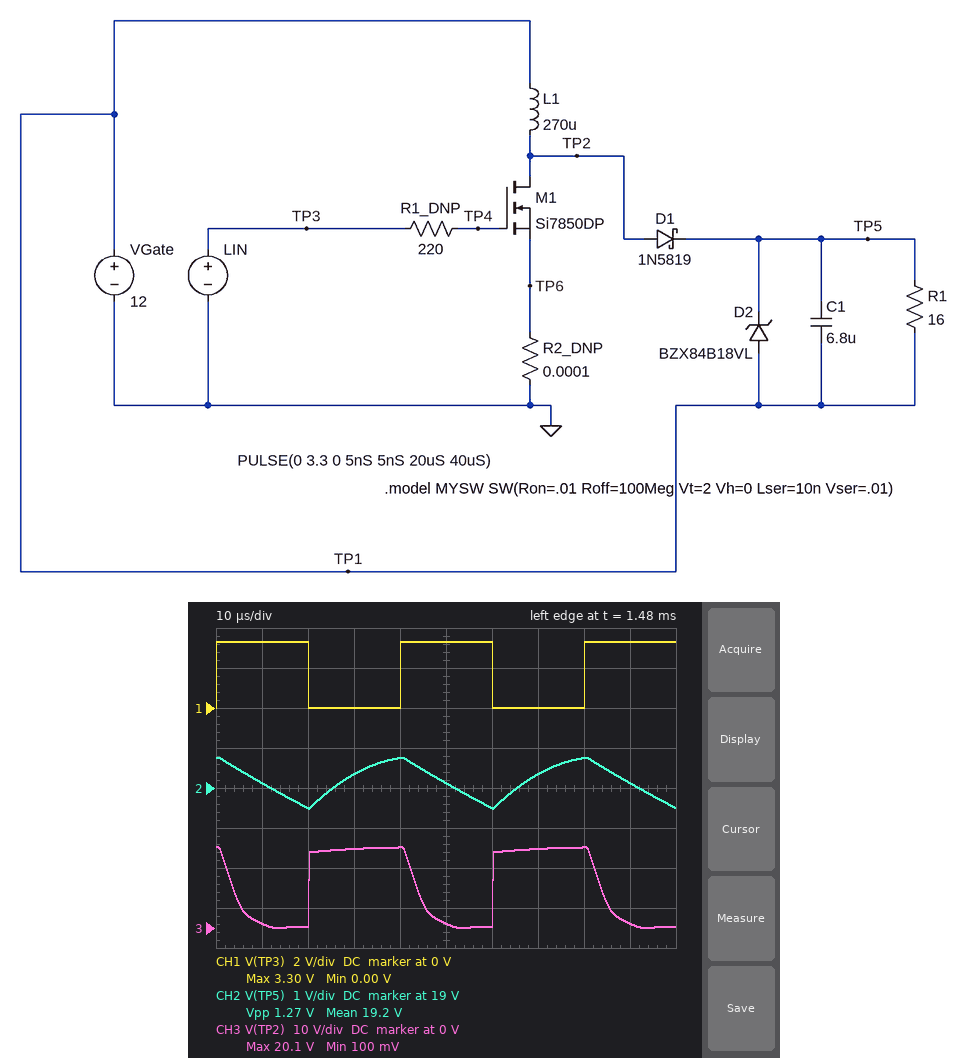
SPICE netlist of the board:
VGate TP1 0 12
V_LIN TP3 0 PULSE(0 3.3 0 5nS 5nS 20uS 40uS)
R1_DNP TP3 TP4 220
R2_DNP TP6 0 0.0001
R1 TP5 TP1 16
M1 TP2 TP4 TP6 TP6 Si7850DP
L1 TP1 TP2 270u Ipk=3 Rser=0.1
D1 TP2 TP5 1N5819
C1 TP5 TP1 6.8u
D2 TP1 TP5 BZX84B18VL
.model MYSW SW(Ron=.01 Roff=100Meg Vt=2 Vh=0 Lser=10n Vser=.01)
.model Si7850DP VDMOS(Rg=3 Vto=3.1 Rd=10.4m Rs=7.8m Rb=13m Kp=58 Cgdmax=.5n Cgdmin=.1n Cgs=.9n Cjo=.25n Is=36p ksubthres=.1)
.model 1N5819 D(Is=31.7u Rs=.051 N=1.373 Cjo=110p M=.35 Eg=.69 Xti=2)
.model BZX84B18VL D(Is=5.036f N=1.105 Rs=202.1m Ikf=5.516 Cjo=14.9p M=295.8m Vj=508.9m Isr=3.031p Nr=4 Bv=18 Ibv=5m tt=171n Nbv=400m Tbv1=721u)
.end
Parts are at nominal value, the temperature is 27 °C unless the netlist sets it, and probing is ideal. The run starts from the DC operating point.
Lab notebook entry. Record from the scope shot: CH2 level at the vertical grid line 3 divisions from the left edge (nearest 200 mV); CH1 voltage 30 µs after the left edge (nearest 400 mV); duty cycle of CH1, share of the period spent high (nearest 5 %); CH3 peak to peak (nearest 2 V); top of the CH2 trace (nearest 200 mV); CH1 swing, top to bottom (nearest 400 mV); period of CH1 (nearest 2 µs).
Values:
19.4 V
0 V
50 %
20 V
19.8 V
3.2 V
40 µs
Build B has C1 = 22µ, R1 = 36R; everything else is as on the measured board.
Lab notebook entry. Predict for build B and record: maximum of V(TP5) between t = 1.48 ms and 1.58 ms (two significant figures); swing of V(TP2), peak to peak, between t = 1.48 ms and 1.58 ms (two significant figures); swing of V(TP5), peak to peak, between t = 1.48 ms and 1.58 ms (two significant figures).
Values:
21 V
22 V
240 mV
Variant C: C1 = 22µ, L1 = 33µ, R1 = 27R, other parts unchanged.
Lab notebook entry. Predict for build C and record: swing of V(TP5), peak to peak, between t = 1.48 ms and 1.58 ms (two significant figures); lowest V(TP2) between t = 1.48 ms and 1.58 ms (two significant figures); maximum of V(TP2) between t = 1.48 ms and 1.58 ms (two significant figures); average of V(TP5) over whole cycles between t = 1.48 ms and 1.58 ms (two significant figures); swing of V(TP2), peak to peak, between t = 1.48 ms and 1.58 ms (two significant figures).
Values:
240 mV
1.5 V
18 V
17 V
16 V
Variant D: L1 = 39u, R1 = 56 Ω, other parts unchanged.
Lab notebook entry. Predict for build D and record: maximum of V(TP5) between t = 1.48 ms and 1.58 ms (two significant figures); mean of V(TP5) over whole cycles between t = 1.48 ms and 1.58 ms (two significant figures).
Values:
21 V
20 V
